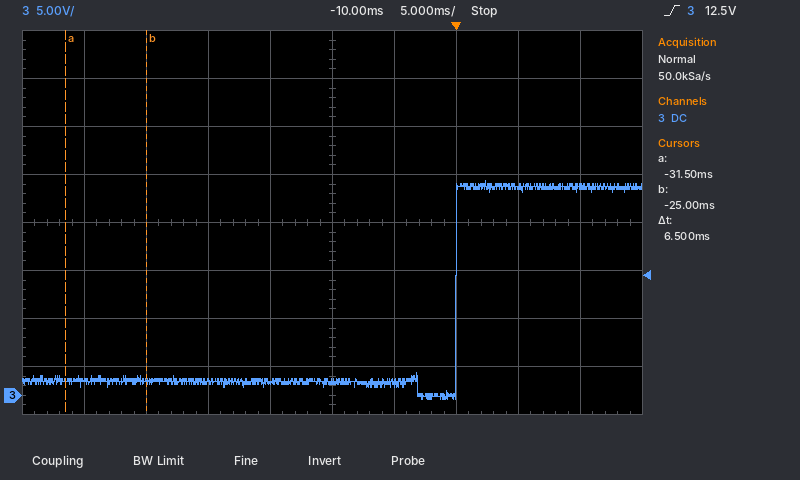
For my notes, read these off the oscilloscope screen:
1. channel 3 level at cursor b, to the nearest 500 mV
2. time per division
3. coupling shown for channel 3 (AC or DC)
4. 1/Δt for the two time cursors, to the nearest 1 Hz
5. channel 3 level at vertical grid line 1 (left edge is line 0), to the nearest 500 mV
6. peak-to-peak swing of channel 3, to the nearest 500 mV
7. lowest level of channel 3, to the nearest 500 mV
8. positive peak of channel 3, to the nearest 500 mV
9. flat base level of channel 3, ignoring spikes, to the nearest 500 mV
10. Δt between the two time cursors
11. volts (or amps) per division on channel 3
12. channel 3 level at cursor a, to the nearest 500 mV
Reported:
1.5 V
5 ms
DC
154 Hz
1.5 V
23.0 V
-500 mV
22.5 V
1.5 V
6.5 ms
5 V
1.5 V
